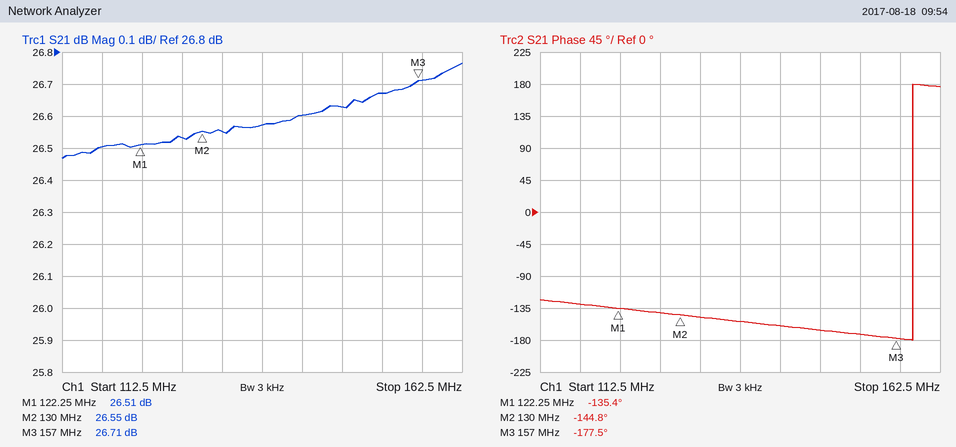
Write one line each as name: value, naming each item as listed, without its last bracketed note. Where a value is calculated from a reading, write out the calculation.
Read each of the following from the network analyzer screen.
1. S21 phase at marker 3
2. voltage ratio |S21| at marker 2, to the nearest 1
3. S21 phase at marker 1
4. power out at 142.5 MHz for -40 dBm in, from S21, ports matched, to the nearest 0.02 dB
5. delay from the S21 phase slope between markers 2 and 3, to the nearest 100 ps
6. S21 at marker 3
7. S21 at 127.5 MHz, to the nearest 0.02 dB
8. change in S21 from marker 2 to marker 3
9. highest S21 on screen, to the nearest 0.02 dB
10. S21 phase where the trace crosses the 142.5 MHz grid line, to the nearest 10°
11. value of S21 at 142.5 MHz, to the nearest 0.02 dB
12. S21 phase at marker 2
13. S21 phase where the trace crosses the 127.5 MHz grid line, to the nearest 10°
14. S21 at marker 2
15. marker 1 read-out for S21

S21 phase at marker 3: -177.5°
voltage ratio |S21| at marker 2, to the nearest 1: 10^(26.55/20) ≈ 21
S21 phase at marker 1: -135.4°
power out at 142.5 MHz for -40 dBm in, from S21, ports matched, to the nearest 0.02 dB: -40 dBm + (26.60 dB) = -13.40 dBm
delay from the S21 phase slope between markers 2 and 3, to the nearest 100 ps: −(-177.5° − (-144.8°))/(360° × 27 MHz) ≈ 3.4 ns
S21 at marker 3: 26.71 dB
S21 at 127.5 MHz, to the nearest 0.02 dB: 26.54 dB
change in S21 from marker 2 to marker 3: 26.71 − (26.55) = 0.16 dB
highest S21 on screen, to the nearest 0.02 dB: 26.76 dB
S21 phase where the trace crosses the 142.5 MHz grid line, to the nearest 10°: -160°
value of S21 at 142.5 MHz, to the nearest 0.02 dB: 26.60 dB
S21 phase at marker 2: -144.8°
S21 phase where the trace crosses the 127.5 MHz grid line, to the nearest 10°: -140°
S21 at marker 2: 26.55 dB
marker 1 read-out for S21: 26.51 dB
